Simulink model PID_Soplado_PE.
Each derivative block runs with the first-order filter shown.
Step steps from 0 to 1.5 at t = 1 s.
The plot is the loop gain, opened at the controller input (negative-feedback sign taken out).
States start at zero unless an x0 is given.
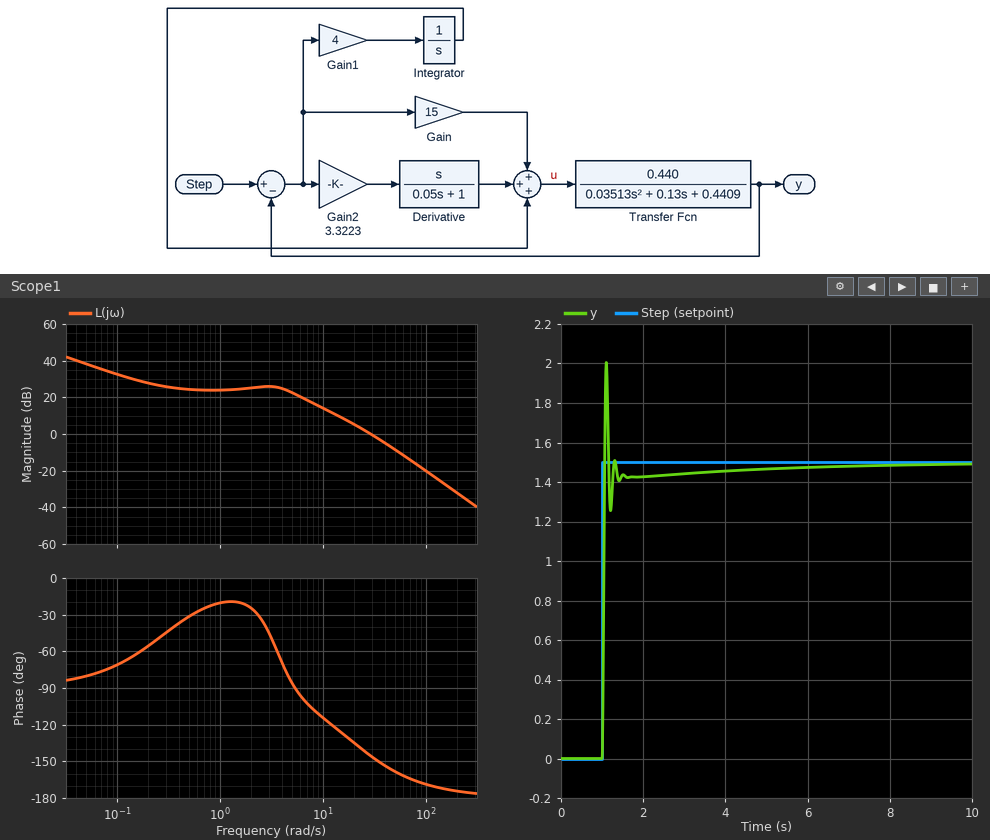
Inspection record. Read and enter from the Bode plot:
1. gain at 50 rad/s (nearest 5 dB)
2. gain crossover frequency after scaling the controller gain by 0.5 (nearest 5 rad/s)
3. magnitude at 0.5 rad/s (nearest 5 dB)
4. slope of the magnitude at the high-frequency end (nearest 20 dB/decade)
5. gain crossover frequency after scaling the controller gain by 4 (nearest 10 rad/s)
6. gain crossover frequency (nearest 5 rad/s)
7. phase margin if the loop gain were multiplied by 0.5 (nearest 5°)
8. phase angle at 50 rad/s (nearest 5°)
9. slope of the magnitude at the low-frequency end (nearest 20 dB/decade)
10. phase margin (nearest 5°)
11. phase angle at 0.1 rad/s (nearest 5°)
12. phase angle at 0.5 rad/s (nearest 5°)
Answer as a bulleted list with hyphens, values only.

- -10 dB
- 20 rad/s
- 25 dB
- -40 dB/decade
- 60 rad/s
- 30 rad/s
- 45°
- -160°
- -20 dB/decade
- 35°
- -70°
- -30°
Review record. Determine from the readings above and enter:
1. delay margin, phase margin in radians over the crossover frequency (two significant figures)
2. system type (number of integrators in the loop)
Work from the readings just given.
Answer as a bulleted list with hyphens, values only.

- 0.020 s
- 1
